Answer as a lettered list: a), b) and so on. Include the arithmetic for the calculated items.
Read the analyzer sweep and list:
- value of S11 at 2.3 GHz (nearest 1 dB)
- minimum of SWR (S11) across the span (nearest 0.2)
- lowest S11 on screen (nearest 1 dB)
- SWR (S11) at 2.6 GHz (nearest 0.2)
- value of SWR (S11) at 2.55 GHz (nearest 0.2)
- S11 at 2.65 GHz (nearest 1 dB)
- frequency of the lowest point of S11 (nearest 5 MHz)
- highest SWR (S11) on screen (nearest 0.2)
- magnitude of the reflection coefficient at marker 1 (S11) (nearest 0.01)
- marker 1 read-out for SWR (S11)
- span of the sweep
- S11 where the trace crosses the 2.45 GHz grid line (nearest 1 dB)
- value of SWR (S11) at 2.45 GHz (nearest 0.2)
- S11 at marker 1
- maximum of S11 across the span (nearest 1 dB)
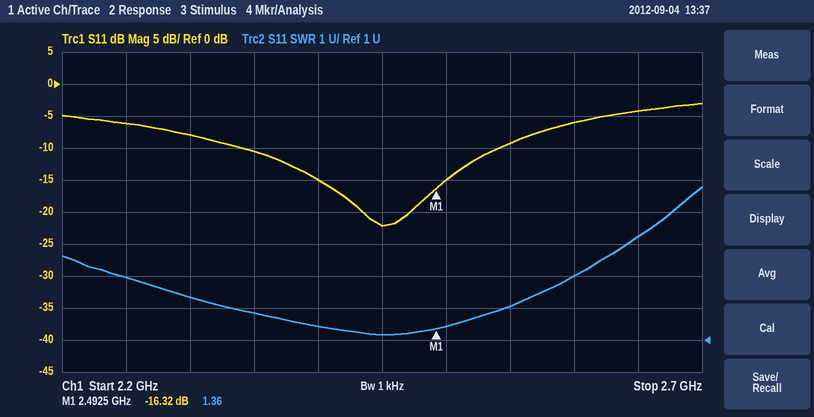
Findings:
a) -8 dB
b) 1.2
c) -22 dB
d) 3.0
e) 2.0
f) -4 dB
g) 2.450 GHz
h) 5.8
i) 10^(-16.32/20) ≈ 0.15
j) 1.36
k) 500 MHz
l) -22 dB
m) 1.2
n) -16.32 dB
o) -3 dB
